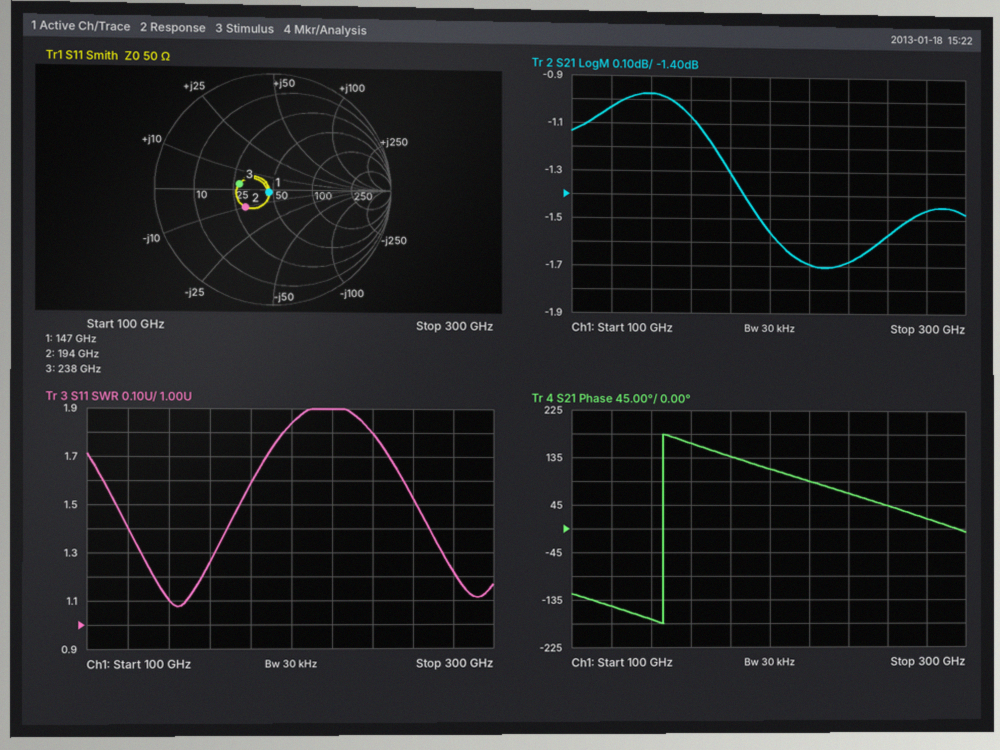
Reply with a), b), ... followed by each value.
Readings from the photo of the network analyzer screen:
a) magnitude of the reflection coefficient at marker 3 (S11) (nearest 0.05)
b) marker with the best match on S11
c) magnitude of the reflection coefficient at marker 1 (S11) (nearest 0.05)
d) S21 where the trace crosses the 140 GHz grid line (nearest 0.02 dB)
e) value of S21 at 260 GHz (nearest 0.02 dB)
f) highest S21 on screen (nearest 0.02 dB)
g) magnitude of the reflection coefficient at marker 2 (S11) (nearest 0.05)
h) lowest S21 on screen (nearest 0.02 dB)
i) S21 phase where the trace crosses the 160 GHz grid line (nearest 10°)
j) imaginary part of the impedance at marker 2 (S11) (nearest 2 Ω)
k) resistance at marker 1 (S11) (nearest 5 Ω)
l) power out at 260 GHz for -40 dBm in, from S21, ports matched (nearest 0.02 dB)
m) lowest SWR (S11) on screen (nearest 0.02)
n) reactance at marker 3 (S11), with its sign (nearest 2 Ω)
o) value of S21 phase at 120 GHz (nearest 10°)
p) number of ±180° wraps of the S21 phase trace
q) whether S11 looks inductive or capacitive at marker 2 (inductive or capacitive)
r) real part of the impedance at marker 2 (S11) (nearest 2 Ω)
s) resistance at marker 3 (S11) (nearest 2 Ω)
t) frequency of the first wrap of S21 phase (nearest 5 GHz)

a) 0.30
b) marker 1
c) 0.05
d) -0.98 dB
e) -1.56 dB
f) -0.98 dB
g) 0.30
h) -1.70 dB
i) 160°
j) -10 Ω
k) 45 Ω
l) -41.56 dBm
m) 1.08
n) +2 Ω
o) -150°
p) 1
q) capacitive
r) 30 Ω
s) 28 Ω
t) 145 GHz
